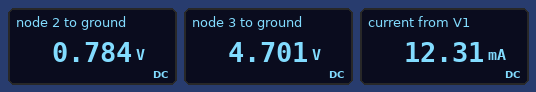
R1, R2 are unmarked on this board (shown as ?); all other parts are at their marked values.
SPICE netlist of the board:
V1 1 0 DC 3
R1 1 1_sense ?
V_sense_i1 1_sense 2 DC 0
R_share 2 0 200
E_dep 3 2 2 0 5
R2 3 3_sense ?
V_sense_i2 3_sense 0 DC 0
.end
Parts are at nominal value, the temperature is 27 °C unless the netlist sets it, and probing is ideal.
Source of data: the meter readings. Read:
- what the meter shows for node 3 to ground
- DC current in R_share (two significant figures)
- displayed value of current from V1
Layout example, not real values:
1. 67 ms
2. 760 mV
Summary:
1. 4.701 V
2. 3.9 mA
3. 12.31 mA
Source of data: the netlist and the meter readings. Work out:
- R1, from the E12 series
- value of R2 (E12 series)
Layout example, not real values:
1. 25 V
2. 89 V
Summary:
1. 180 Ω
2. 560 Ω
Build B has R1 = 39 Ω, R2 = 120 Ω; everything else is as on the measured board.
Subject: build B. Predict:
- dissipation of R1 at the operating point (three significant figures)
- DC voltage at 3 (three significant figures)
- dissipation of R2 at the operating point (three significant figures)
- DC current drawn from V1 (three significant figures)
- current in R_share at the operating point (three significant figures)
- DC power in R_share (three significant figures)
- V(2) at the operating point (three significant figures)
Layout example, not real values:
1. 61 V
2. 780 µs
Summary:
1. 107 mW
2. 5.72 V
3. 273 mW
4. 52.5 mA
5. 4.77 mA
6. 4.55 mW
7. 954 mV
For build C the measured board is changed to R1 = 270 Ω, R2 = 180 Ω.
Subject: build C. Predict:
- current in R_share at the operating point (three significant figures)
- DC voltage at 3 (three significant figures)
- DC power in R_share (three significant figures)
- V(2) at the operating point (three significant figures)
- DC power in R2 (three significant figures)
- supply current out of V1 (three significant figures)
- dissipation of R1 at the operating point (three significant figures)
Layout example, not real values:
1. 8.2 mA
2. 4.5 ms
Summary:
1. 1.32 mA
2. 1.59 V
3. 349 µW
4. 264 mV
5. 14.0 mW
6. 10.1 mA
7. 27.7 mW
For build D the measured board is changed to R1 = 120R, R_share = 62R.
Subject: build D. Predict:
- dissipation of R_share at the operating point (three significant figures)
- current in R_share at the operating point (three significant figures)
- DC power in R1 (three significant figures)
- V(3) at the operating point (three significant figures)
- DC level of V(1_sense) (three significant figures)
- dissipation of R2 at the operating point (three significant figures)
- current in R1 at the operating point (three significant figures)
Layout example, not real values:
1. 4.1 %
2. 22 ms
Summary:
1. 8.15 mW
2. 11.5 mA
3. 43.7 mW
4. 4.26 V
5. 711 mV
6. 32.5 mW
7. 19.1 mA
